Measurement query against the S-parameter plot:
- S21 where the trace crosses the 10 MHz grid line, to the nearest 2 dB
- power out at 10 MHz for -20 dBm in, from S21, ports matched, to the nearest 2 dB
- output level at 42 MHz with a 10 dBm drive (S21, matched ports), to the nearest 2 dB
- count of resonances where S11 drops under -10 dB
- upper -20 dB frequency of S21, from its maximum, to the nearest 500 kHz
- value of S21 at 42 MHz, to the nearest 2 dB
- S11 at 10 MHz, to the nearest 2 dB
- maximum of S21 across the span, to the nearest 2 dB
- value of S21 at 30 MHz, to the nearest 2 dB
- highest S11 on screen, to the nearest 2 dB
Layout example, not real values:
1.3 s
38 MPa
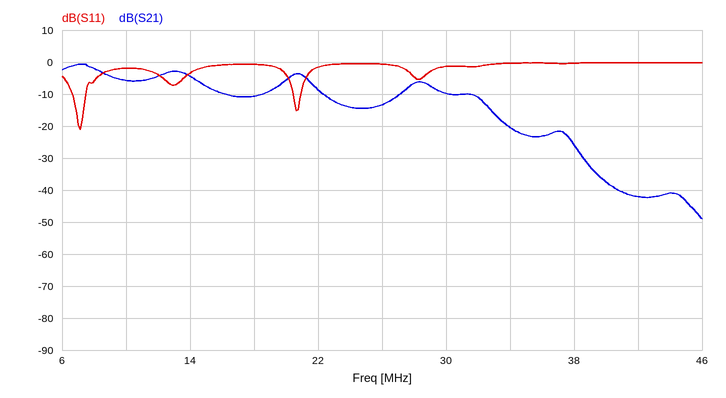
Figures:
-6 dB
-26 dBm
-32 dBm
2
34.0 MHz
-42 dB
-2 dB
0 dB
-10 dB
0 dB
